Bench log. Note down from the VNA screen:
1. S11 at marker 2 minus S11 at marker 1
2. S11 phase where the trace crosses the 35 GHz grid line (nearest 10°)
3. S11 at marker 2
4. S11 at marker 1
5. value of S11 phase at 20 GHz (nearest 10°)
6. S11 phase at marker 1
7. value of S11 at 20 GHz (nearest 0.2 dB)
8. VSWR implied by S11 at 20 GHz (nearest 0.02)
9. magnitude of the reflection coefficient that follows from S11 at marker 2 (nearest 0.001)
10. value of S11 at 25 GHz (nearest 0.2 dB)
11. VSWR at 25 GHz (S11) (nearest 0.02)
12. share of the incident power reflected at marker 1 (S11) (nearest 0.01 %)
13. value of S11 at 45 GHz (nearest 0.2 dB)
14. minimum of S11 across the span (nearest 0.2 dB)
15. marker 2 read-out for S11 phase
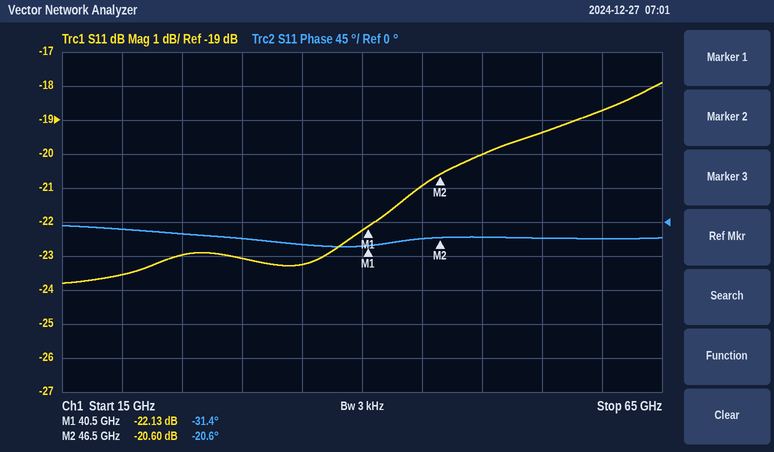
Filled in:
1.53 dB
-30°
-20.60 dB
-22.13 dB
-10°
-31.4°
-23.6 dB
1.14
0.093
-23.0 dB
1.16
0.61 %
-21.0 dB
-23.8 dB
-20.6°
